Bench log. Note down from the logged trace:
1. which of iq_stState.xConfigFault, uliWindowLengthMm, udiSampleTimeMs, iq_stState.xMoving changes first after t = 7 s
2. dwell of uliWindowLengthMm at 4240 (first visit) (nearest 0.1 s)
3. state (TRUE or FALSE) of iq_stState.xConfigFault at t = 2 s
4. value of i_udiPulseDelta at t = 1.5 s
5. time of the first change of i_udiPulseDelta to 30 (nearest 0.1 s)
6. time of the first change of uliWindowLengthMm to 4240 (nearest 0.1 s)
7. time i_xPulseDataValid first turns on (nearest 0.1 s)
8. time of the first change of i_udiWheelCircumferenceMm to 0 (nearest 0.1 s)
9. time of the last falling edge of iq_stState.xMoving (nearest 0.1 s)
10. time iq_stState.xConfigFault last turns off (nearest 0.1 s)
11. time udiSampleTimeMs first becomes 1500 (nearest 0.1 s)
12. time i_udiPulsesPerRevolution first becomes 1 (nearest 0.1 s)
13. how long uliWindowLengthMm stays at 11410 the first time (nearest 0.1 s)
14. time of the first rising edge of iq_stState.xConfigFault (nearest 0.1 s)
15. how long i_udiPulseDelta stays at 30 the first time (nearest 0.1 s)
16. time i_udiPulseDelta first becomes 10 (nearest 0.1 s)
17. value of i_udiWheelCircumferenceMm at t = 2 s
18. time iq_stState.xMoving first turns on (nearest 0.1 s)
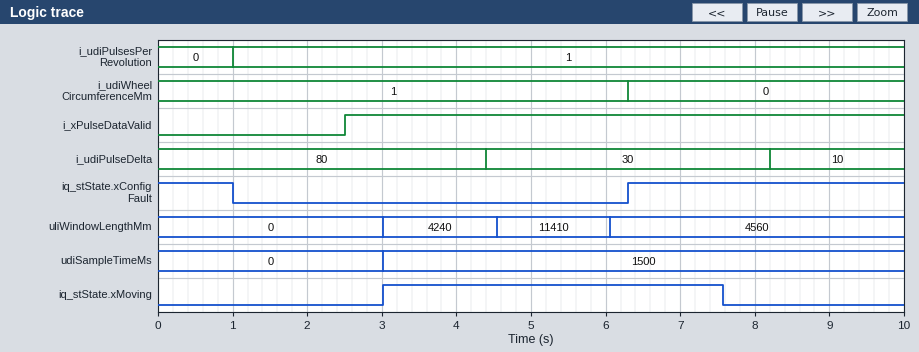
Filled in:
iq_stState.xMoving
1.5 s
FALSE
80
4.4 s
3.0 s
2.5 s
6.3 s
7.6 s
1.0 s
3.0 s
1.0 s
1.5 s
6.3 s
3.8 s
8.2 s
1
3.0 s
